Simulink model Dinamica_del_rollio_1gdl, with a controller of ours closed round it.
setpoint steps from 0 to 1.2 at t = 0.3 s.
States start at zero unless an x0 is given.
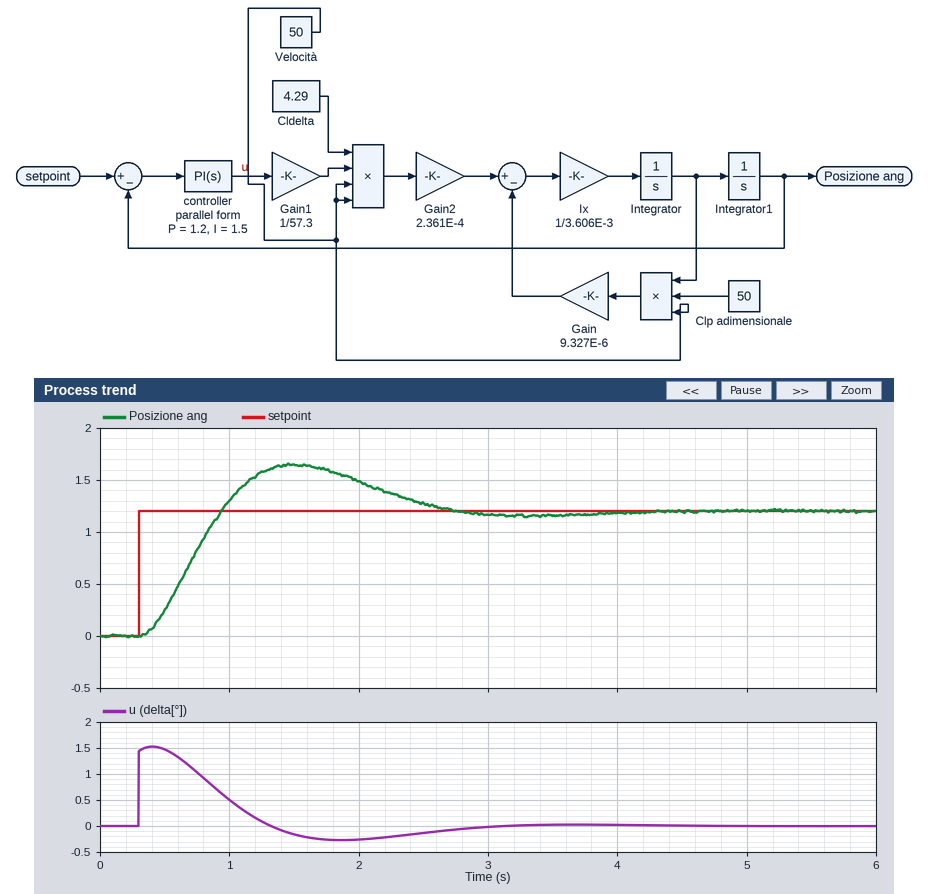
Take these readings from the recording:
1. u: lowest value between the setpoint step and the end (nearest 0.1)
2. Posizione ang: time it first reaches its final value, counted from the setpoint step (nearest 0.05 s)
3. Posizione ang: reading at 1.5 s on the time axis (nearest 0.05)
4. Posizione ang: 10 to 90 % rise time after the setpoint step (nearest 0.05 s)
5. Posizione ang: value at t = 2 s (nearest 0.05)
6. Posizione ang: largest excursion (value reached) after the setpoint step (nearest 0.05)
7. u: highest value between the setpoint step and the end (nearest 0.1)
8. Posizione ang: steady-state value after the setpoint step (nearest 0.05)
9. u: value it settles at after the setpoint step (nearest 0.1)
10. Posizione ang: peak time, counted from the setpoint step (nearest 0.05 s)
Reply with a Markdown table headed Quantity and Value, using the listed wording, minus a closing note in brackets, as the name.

| Quantity | Value |
|---|---|
| u: lowest value between the setpoint step and the end | -0.3 |
| Posizione ang: time it first reaches its final value, counted from the setpoint step | 0.65 s |
| Posizione ang: reading at 1.5 s on the time axis | 1.65 |
| Posizione ang: 10 to 90 % rise time after the setpoint step | 0.45 s |
| Posizione ang: value at t = 2 s | 1.50 |
| Posizione ang: largest excursion (value reached) after the setpoint step | 1.65 |
| u: highest value between the setpoint step and the end | 1.5 |
| Posizione ang: steady-state value after the setpoint step | 1.20 |
| u: value it settles at after the setpoint step | 0.0 |
| Posizione ang: peak time, counted from the setpoint step | 1.20 s |
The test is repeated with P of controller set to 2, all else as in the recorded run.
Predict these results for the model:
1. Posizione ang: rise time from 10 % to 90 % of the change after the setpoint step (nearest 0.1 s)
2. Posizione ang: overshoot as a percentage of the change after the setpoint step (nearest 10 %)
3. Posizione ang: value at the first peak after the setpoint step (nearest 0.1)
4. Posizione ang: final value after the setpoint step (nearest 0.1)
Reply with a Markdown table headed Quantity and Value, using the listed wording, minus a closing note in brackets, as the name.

| Quantity | Value |
|---|---|
| Posizione ang: rise time from 10 % to 90 % of the change after the setpoint step | 0.3 s |
| Posizione ang: overshoot as a percentage of the change after the setpoint step | 30 % |
| Posizione ang: value at the first peak after the setpoint step | 1.5 |
| Posizione ang: final value after the setpoint step | 1.2 |
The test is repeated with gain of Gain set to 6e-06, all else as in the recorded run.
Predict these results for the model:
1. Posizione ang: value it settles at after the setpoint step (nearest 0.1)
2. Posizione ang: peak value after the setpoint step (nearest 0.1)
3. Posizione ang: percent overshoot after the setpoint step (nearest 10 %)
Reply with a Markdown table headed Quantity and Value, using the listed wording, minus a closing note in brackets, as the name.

| Quantity | Value |
|---|---|
| Posizione ang: value it settles at after the setpoint step | 1.2 |
| Posizione ang: peak value after the setpoint step | 1.8 |
| Posizione ang: percent overshoot after the setpoint step | 50 % |
